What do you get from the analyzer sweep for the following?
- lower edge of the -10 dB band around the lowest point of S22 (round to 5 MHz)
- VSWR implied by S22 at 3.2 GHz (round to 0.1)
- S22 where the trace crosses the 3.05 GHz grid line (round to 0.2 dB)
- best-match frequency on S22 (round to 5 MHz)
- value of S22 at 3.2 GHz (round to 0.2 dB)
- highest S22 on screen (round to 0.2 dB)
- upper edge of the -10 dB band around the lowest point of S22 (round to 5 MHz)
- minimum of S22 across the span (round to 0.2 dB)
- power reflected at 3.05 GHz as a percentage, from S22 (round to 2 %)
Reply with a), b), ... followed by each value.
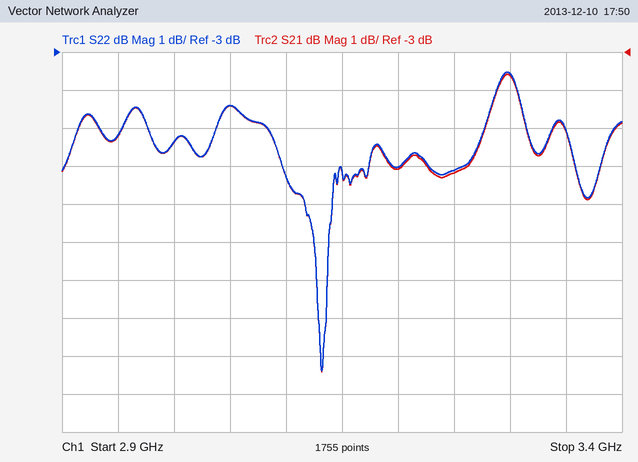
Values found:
a) 3.130 GHz
b) 3.0
c) -4.4 dB
d) 3.130 GHz
e) -6.0 dB
f) -3.6 dB
g) 3.135 GHz
h) -11.4 dB
i) 36 %
